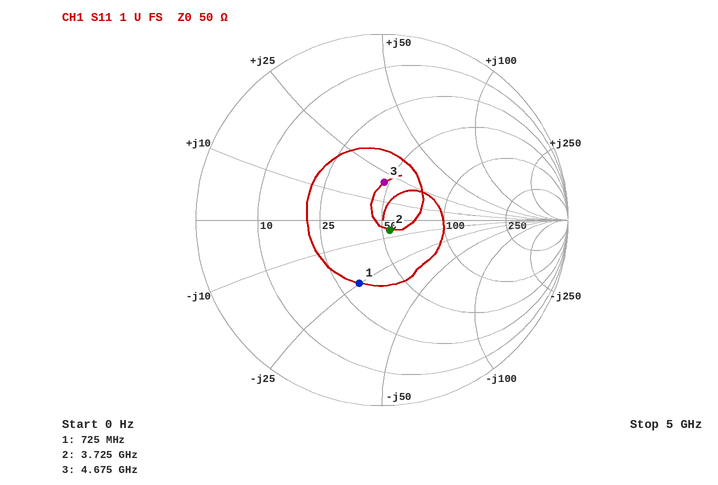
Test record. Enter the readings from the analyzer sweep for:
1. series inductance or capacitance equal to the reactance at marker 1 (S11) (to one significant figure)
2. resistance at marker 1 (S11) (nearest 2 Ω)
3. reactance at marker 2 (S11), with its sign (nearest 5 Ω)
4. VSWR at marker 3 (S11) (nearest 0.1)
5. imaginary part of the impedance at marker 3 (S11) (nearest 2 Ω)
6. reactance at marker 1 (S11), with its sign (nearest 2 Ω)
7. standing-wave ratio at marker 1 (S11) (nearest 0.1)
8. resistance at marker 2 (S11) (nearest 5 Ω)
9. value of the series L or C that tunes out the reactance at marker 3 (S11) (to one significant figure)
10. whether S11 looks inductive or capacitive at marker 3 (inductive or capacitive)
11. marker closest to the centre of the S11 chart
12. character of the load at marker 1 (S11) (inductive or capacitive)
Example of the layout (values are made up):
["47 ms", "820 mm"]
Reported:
["9 pF", "32 Ω", "-5 Ω", "1.5", "+20 Ω", "-24 Ω", "2.1", "55 Ω", "2 pF", "inductive", "marker 2", "capacitive"]
